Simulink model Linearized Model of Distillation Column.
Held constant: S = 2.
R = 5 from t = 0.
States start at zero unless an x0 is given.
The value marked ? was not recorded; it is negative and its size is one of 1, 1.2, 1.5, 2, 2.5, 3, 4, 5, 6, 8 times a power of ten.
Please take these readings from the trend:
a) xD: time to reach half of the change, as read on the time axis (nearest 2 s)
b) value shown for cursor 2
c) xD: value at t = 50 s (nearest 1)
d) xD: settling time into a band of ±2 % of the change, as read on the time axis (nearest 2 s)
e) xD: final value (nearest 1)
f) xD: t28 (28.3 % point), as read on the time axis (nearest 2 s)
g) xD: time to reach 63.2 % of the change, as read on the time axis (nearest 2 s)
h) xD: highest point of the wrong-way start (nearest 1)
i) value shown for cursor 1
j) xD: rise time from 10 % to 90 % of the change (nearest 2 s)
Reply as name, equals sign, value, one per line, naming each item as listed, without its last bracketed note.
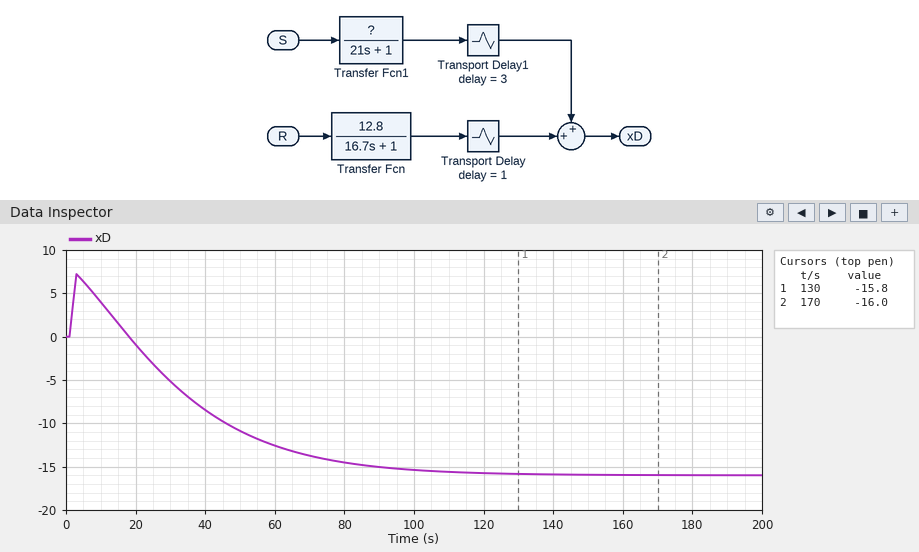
xD: time to reach half of the change, as read on the time axis = 38 s
value shown for cursor 2 = -16.0
xD: value at t = 50 s = -11
xD: settling time into a band of ±2 % of the change, as read on the time axis = 114 s
xD: final value = -16
xD: t28 (28.3 % point), as read on the time axis = 28 s
xD: time to reach 63.2 % of the change, as read on the time axis = 46 s
xD: highest point of the wrong-way start = 7
value shown for cursor 1 = -15.8
xD: rise time from 10 % to 90 % of the change = 56 s
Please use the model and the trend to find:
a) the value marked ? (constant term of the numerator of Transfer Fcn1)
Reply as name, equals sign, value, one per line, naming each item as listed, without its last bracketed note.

the value marked ? = -40
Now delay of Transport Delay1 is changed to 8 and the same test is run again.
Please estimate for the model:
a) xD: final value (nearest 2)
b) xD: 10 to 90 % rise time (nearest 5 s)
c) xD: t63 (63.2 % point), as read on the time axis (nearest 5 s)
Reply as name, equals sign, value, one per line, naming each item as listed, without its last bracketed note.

xD: final value = -16
xD: 10 to 90 % rise time = 50 s
xD: t63 (63.2 % point), as read on the time axis = 55 s
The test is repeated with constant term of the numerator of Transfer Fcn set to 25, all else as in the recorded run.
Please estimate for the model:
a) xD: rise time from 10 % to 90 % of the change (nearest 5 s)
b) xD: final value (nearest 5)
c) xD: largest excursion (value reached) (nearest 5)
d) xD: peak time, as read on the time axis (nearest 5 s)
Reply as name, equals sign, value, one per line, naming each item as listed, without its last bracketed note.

xD: rise time from 10 % to 90 % of the change = 20 s
xD: final value = 45
xD: largest excursion (value reached) = 45
xD: peak time, as read on the time axis = 50 s
